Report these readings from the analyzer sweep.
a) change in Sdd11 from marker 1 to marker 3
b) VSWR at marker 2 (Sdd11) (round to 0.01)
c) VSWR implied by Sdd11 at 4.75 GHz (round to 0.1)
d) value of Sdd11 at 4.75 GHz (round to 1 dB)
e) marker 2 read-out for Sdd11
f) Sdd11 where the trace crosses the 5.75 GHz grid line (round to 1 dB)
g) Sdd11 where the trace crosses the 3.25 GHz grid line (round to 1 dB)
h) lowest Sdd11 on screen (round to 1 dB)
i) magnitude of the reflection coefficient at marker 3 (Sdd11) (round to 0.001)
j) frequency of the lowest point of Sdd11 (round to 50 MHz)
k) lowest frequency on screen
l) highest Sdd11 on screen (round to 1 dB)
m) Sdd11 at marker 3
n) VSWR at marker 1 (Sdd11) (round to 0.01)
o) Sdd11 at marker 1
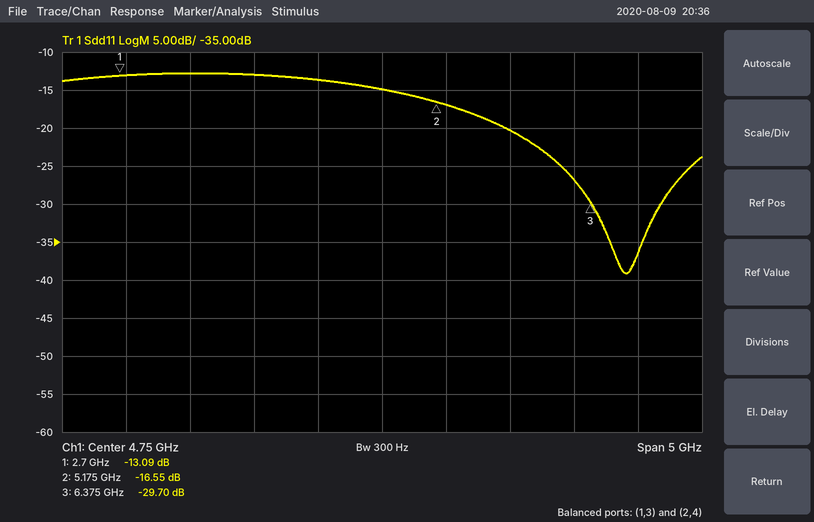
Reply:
-16.61 dB
1.35
1.4
-15 dB
-16.55 dB
-20 dB
-13 dB
-39 dB
0.033
6.65 GHz
2.25 GHz
-13 dB
-29.70 dB
1.57
-13.09 dB
